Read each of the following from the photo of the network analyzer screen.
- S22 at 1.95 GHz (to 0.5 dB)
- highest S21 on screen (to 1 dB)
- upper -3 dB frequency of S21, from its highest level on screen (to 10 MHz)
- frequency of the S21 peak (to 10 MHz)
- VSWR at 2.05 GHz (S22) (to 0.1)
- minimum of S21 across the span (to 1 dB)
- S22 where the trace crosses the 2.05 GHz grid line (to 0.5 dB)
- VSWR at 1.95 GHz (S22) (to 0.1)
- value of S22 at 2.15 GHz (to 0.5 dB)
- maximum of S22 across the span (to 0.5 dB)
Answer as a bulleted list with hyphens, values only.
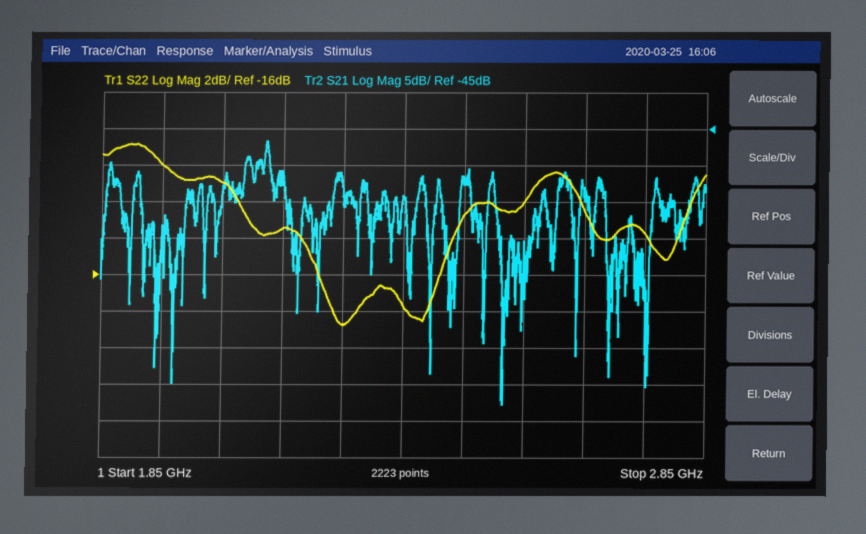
- -10.0 dB
- -47 dB
- 2.13 GHz
- 2.12 GHz
- 1.8
- -83 dB
- -11.0 dB
- 1.9
- -13.5 dB
- -9.0 dB
